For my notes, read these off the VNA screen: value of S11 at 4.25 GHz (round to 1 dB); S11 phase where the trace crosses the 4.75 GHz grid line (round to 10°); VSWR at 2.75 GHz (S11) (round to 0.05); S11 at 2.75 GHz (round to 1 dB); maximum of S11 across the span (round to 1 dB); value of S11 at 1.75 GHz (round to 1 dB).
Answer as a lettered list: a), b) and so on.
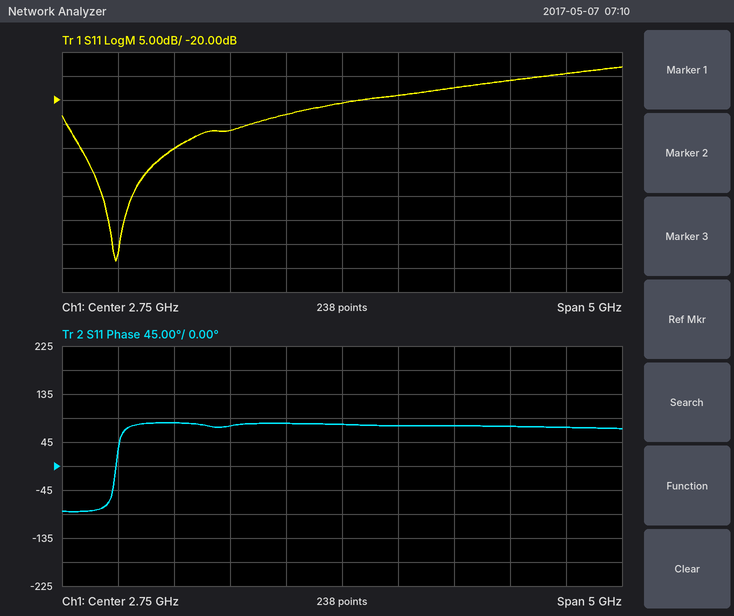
a) -16 dB
b) 70°
c) 1.20
d) -21 dB
e) -13 dB
f) -26 dB
